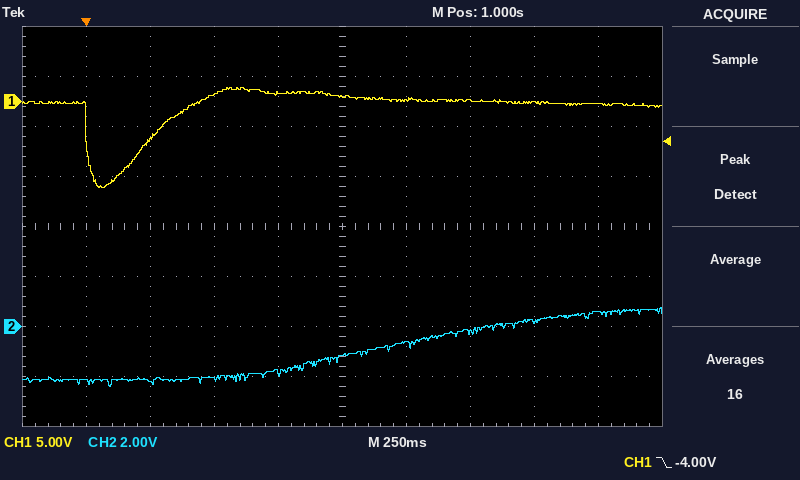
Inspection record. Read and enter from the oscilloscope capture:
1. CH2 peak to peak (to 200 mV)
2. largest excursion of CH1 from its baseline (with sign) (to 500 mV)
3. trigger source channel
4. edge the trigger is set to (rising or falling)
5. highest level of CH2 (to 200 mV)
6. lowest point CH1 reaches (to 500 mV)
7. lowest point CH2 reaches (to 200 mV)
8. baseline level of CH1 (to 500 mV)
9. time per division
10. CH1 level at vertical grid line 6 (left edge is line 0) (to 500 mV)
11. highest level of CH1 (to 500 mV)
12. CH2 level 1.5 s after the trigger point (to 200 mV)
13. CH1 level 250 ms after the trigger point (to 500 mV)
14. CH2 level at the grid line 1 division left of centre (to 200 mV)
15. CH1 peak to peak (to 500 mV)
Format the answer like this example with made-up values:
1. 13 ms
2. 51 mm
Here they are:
1. 3.2 V
2. -8.5 V
3. CH1
4. falling
5. 800 mV
6. -8.5 V
7. -2.4 V
8. 0.0 V
9. 250 ms
10. 0.0 V
11. 1.5 V
12. -200 mV
13. -3.5 V
14. -1.8 V
15. 10.0 V
